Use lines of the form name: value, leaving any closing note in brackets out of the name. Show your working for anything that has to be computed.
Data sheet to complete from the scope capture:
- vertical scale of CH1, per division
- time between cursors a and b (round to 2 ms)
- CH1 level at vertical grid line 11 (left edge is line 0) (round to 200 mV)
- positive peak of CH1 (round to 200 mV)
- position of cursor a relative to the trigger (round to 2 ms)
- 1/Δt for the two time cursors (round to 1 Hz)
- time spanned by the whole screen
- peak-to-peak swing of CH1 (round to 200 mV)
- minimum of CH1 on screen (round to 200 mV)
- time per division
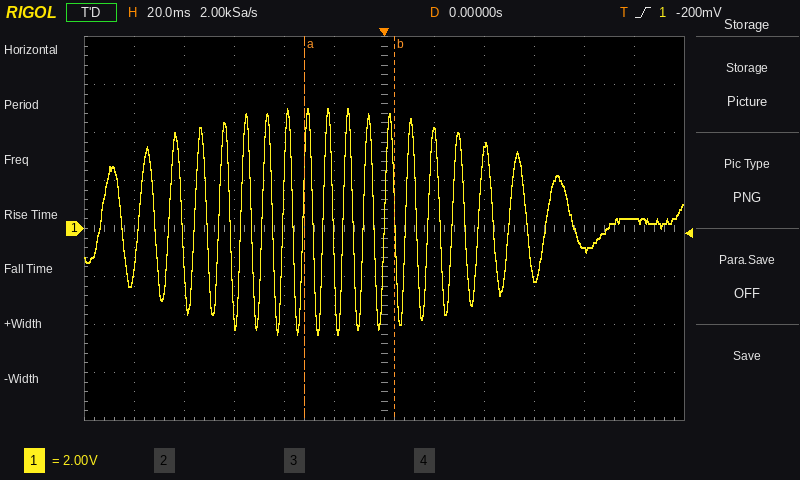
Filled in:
vertical scale of CH1, per division: 2 V
time between cursors a and b: 36 ms
CH1 level at vertical grid line 11 (left edge is line 0): 400 mV
positive peak of CH1: 5.0 V
position of cursor a relative to the trigger: -32 ms
1/Δt for the two time cursors: 1 / 36 ms ≈ 28 Hz
time spanned by the whole screen: 240 ms
peak-to-peak swing of CH1: 5.0 V − (-4.4 V) = 9.4 V
minimum of CH1 on screen: -4.4 V
time per division: 20 ms
